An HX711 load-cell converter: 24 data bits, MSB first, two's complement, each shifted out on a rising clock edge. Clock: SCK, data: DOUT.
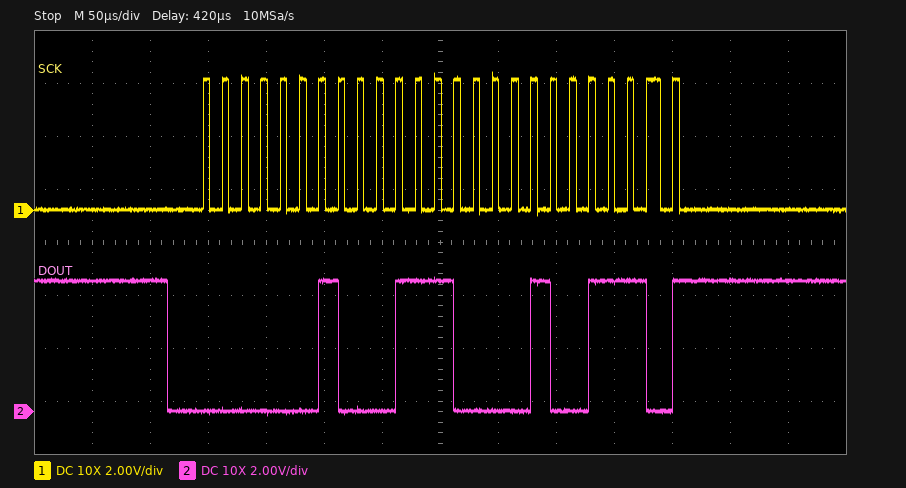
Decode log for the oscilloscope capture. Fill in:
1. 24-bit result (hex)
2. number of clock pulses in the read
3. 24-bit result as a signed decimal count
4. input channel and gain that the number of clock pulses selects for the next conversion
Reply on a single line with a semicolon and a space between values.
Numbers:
0x02384E; 25; 145486; channel A, gain 128
